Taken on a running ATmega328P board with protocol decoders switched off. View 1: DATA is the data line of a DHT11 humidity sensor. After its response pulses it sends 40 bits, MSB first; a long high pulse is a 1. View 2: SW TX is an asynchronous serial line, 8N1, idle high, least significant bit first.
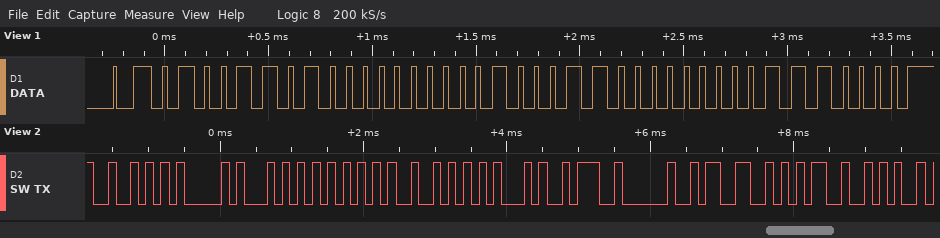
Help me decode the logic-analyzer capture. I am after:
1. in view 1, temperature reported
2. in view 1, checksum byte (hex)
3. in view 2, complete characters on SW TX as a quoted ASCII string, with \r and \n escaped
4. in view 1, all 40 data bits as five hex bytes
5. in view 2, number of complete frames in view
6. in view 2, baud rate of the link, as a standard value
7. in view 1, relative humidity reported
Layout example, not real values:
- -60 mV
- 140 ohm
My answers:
- 35.0 °C
- 0x70
- "RATURE: 35*"
- 4D 00 23 00 70
- 11
- 9600 baud
- 77 %
